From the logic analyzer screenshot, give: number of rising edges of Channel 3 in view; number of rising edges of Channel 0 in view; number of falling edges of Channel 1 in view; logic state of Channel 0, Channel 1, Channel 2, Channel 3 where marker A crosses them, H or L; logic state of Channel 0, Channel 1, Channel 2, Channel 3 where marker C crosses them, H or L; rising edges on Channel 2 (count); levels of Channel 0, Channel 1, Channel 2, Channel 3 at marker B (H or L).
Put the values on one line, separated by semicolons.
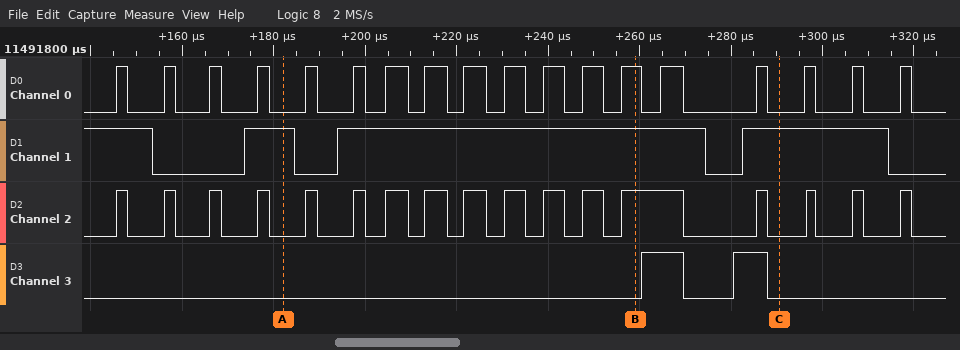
2; 18; 4; Channel 0=L, Channel 1=H, Channel 2=L, Channel 3=L; Channel 0=L, Channel 1=H, Channel 2=L, Channel 3=L; 17; Channel 0=H, Channel 1=H, Channel 2=H, Channel 3=L
